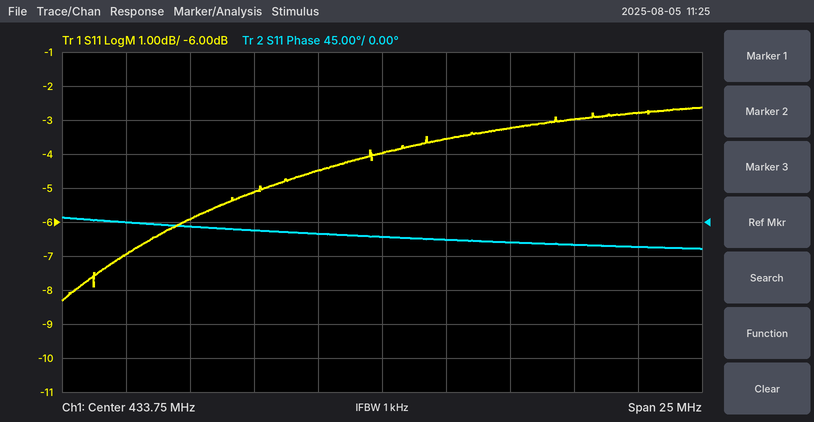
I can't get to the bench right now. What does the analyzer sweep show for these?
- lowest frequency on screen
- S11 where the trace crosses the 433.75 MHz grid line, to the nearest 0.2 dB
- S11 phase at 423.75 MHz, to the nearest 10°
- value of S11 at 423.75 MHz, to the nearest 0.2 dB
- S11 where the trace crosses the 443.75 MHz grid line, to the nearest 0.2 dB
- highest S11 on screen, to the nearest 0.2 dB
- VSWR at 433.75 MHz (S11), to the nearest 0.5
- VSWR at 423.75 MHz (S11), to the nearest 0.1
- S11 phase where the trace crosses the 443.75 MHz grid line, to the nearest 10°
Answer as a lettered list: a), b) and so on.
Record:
a) 421.25 MHz
b) -4.0 dB
c) 0°
d) -7.0 dB
e) -2.8 dB
f) -2.6 dB
g) 4.5
h) 2.6
i) -30°
